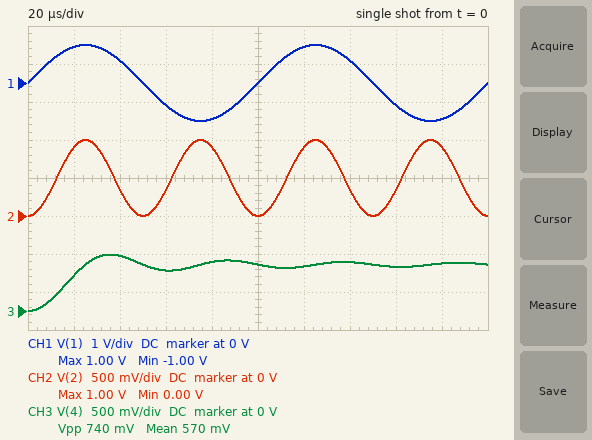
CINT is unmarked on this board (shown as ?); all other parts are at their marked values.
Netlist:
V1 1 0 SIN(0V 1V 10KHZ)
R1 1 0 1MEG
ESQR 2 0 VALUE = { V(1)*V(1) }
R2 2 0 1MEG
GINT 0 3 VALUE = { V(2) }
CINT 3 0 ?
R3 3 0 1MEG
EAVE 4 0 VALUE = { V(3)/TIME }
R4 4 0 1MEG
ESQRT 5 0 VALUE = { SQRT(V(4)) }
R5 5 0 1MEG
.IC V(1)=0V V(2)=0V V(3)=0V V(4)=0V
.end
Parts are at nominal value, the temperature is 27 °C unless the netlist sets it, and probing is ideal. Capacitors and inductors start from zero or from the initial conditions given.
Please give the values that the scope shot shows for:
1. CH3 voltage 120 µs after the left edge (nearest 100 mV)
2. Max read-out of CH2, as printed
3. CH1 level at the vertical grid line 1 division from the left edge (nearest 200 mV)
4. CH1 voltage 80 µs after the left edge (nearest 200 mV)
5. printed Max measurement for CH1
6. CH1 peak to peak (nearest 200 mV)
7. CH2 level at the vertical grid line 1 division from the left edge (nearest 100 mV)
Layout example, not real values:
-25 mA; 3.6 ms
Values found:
600 mV; 1.00 V; 1.0 V; -1.0 V; 1.00 V; 2.0 V; 900 mV
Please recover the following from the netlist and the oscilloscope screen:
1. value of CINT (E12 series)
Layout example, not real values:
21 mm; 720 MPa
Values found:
820 mF
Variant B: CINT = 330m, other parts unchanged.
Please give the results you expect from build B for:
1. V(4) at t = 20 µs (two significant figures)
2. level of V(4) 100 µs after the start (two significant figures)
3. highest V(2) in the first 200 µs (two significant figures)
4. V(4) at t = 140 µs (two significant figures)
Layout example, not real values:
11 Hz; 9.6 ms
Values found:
1.2 V; 1.5 V; 1.0 V; 1.6 V
